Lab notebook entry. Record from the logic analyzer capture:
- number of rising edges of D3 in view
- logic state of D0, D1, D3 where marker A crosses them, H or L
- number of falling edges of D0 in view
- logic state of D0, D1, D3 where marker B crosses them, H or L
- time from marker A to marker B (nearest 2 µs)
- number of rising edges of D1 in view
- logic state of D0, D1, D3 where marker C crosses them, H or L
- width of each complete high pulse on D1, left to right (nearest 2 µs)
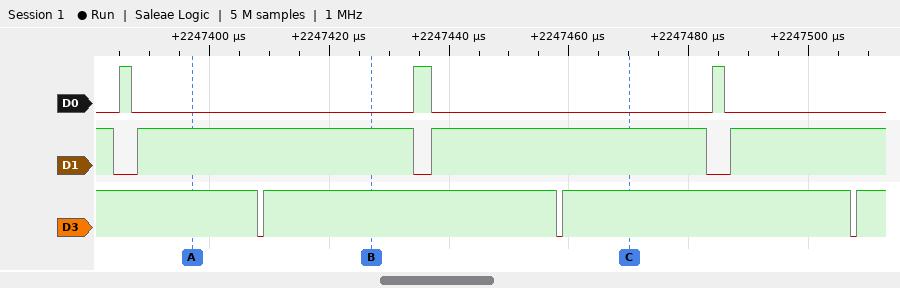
3
D0=L, D1=H, D3=H
3
D0=L, D1=H, D3=H
30 µs
3
D0=L, D1=H, D3=H
46 µs, 46 µs
